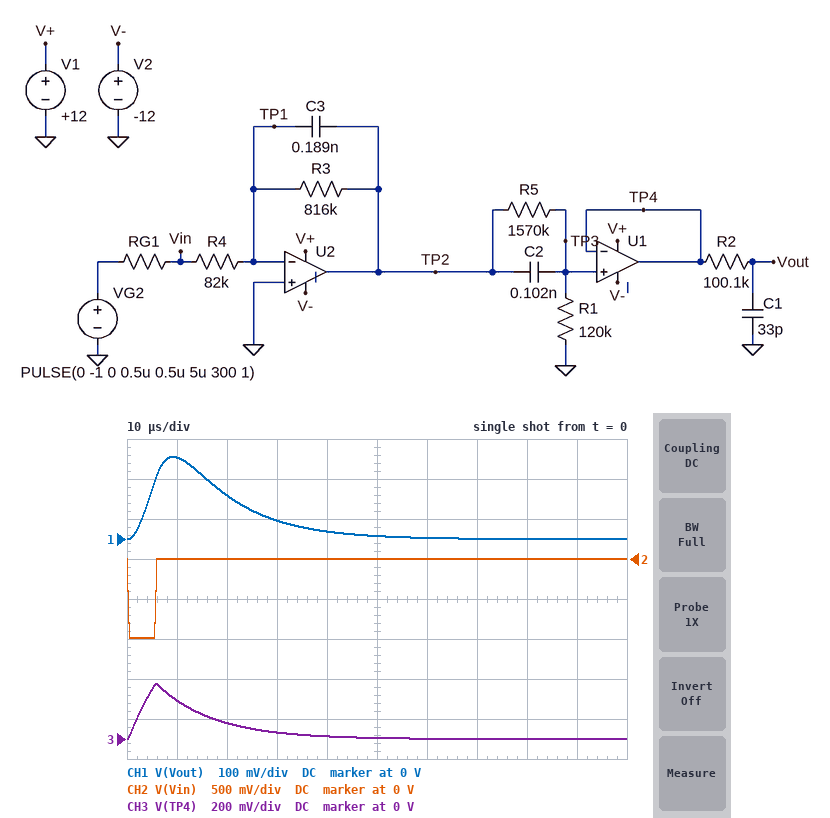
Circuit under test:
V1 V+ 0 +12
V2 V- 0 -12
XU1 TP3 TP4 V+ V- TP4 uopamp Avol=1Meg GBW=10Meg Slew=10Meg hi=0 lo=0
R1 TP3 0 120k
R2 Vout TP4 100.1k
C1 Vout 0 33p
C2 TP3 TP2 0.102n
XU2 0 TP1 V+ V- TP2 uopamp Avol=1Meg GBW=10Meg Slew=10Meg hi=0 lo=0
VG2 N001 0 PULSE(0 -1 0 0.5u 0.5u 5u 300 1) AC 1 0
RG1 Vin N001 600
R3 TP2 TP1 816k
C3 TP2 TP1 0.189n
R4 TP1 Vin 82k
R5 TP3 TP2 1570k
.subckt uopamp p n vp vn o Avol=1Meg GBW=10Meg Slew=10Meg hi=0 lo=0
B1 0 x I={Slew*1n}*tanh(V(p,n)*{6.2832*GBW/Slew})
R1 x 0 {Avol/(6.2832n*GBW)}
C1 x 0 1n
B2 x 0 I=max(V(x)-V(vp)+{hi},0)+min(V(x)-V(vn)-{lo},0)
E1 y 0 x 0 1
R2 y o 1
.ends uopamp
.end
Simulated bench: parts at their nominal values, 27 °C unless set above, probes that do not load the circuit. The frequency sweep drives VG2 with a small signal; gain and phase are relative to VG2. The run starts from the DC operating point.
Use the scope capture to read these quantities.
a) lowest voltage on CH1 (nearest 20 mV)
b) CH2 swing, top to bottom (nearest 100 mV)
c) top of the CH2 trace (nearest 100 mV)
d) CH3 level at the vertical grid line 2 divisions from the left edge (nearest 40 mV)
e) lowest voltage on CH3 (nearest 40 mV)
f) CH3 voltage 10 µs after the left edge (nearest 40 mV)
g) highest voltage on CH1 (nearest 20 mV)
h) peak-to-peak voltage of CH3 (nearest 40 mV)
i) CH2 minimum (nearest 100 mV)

0 V
1.0 V
0 V
80 mV
0 V
200 mV
200 mV
280 mV
-1.0 V
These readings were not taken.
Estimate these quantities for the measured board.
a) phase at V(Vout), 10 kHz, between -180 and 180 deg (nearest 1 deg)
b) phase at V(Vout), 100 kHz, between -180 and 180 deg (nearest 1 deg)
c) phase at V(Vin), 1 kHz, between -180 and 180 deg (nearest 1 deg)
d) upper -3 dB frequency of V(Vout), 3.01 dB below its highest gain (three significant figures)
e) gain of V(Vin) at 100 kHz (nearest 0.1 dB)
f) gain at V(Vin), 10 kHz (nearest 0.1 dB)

133 deg
33 deg
0 deg
13.4 kHz
-0.1 dB
-0.1 dB
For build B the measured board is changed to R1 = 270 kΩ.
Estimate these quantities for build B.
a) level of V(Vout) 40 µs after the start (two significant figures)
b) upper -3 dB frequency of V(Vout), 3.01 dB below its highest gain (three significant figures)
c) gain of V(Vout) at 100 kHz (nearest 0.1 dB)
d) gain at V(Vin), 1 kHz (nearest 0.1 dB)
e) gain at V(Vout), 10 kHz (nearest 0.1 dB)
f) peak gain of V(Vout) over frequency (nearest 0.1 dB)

84 mV
7.02 kHz
-27.1 dB
-0.1 dB
-1.7 dB
3.3 dB
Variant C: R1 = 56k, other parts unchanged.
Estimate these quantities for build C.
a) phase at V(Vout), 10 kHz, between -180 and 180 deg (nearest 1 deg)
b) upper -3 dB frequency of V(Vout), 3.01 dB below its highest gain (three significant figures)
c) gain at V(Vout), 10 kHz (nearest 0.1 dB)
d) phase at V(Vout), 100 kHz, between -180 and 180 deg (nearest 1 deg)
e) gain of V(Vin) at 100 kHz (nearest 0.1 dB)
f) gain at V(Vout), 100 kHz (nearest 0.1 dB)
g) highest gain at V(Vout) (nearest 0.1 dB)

149 deg
23.3 kHz
-9.7 dB
41 deg
-0.1 dB
-27.4 dB
-9.1 dB
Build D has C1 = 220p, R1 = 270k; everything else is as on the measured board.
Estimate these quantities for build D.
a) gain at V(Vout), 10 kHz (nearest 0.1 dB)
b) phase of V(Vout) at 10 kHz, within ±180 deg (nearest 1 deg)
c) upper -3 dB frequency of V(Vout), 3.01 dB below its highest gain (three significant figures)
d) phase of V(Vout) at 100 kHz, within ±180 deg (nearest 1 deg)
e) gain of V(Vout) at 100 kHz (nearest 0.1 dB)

-6.1 dB
70 deg
4.75 kHz
7 deg
-42.7 dB
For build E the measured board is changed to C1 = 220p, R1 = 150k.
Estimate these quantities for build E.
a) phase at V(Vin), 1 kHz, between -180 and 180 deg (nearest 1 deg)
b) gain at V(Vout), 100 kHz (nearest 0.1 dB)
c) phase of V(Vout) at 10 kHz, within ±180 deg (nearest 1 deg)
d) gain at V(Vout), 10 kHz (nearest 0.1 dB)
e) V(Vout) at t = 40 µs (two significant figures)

0 deg
-42.7 dB
85 deg
-8.1 dB
70 mV
